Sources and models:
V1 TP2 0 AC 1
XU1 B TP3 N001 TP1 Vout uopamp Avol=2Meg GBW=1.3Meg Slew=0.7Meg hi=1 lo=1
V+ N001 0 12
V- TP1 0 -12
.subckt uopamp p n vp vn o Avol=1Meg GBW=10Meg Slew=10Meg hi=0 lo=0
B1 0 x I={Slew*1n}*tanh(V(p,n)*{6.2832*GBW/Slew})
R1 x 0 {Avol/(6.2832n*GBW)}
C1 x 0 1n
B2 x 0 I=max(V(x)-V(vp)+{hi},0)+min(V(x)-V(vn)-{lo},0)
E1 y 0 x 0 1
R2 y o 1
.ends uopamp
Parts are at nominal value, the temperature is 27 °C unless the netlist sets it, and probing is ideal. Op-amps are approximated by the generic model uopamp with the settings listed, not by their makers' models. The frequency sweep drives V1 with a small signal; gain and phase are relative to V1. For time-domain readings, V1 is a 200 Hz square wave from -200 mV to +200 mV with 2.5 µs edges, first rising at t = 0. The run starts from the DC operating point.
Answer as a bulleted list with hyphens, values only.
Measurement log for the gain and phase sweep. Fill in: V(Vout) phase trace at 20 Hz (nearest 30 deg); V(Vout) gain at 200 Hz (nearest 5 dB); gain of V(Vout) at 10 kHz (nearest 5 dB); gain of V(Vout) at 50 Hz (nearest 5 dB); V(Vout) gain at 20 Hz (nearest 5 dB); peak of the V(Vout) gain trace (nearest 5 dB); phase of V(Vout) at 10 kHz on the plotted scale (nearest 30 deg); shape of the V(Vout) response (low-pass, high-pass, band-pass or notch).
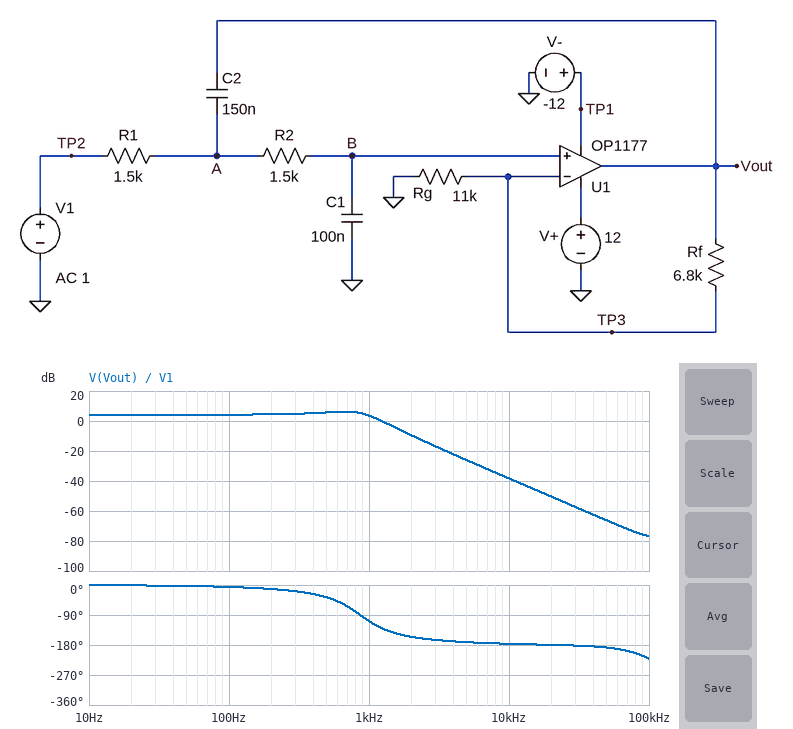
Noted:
- 0 deg
- 5 dB
- -40 dB
- 5 dB
- 5 dB
- 5 dB
- -180 deg
- low-pass
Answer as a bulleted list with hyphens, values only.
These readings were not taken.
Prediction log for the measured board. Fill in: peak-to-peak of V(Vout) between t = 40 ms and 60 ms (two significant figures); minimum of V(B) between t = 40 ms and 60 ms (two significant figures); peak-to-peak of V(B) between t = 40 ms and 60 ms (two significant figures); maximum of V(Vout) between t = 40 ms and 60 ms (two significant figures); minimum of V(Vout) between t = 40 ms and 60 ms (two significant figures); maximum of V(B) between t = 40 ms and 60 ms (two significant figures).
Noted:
- 930 mV
- -290 mV
- 570 mV
- 460 mV
- -460 mV
- 290 mV
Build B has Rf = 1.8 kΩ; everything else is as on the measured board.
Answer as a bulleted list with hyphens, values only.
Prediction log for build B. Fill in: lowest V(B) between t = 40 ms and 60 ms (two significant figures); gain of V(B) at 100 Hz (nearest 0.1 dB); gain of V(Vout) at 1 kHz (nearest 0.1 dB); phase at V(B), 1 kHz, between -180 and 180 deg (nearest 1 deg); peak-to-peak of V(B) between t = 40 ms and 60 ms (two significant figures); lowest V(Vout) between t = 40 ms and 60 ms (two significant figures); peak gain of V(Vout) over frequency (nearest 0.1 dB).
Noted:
- -220 mV
- 0 dB
- -3.2 dB
- -101 deg
- 430 mV
- -250 mV
- 1.3 dB
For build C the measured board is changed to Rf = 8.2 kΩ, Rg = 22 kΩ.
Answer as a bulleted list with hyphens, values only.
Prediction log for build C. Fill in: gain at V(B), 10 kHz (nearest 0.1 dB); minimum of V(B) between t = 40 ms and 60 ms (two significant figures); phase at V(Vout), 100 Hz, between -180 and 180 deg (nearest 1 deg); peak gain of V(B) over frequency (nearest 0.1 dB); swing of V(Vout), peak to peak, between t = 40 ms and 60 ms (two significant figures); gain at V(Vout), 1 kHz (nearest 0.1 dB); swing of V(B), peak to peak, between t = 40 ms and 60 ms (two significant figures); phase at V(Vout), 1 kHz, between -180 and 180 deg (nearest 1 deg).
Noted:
- -42.5 dB
- -240 mV
- -8 deg
- 0.4 dB
- 660 mV
- -0.2 dB
- 480 mV
- -104 deg
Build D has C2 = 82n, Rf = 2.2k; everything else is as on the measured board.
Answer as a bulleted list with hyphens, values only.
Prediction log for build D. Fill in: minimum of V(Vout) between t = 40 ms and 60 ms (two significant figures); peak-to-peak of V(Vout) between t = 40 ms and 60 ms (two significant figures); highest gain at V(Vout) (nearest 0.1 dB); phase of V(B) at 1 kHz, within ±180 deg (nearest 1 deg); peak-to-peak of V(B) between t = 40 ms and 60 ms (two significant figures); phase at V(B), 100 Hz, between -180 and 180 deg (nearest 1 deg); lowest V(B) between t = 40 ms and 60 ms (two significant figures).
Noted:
- -240 mV
- 480 mV
- 1.6 dB
- -81 deg
- 400 mV
- -10 deg
- -200 mV
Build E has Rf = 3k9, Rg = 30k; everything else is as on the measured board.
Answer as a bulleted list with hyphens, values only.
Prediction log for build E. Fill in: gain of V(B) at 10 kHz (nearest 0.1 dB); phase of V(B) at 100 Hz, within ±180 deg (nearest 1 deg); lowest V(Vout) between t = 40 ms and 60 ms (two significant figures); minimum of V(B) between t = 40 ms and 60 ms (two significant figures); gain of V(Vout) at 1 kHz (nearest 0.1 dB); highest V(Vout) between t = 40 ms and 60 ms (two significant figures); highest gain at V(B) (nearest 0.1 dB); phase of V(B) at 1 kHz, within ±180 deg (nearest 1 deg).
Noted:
- -42.5 dB
- -10 deg
- -240 mV
- -210 mV
- -3.7 dB
- 240 mV
- 0 dB
- -101 deg
